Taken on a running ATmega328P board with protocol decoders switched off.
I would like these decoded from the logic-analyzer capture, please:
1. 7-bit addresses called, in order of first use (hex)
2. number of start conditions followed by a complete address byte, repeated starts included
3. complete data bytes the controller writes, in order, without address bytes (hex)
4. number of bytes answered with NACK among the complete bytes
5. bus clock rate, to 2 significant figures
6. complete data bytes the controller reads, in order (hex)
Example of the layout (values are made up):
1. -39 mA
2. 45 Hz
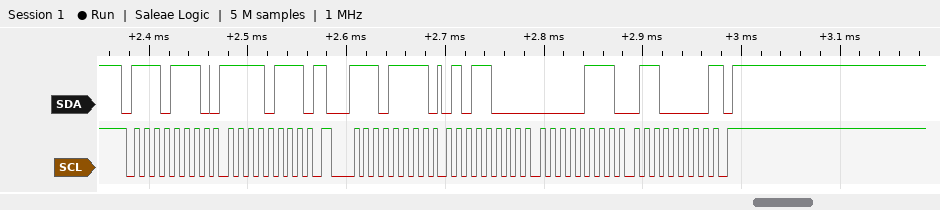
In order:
1. 0x77
2. 2
3. F7
4. 1
5. 100 kHz
6. 58 07 60
